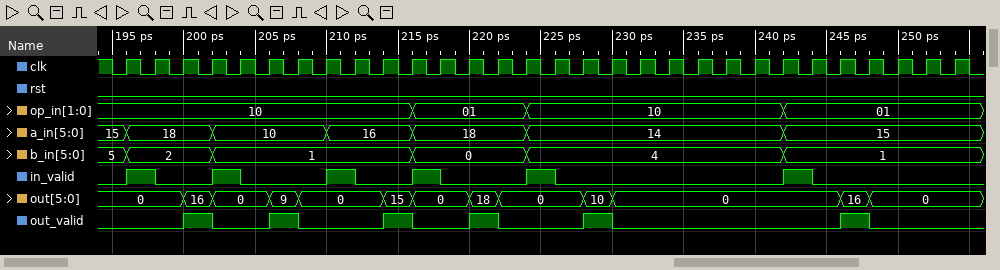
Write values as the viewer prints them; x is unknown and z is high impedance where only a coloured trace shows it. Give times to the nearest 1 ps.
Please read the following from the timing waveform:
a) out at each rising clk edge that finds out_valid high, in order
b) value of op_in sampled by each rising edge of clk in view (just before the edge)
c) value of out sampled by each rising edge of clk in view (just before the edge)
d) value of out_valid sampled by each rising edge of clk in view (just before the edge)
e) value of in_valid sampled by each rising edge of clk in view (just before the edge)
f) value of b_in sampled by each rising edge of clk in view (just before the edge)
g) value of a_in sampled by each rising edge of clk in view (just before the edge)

16, 9, 15, 18, 10, 16
10, 10, 10, 10, 10, 10, 10, 10, 10, 10, 10, 01, 01, 01, 01, 10, 10, 10, 10, 10, 10, 10, 10, 10, 01, 01, 01, 01, 01, 01
0, 0, 0, 16, 0, 0, 9, 0, 0, 0, 15, 0, 0, 18, 0, 0, 0, 10, 0, 0, 0, 0, 0, 0, 0, 0, 16, 0, 0, 0
0 0 0 1 0 0 1 0 0 0 1 0 0 1 0 0 0 1 0 0 0 0 0 0 0 0 1 0 0 0
0 1 0 0 1 0 0 0 1 0 0 1 0 0 0 1 0 0 0 0 0 0 0 0 1 0 0 0 0 0
5, 2, 2, 2, 1, 1, 1, 1, 1, 1, 1, 0, 0, 0, 0, 4, 4, 4, 4, 4, 4, 4, 4, 4, 1, 1, 1, 1, 1, 1
15, 18, 18, 18, 10, 10, 10, 10, 16, 16, 16, 18, 18, 18, 18, 14, 14, 14, 14, 14, 14, 14, 14, 14, 15, 15, 15, 15, 15, 15
